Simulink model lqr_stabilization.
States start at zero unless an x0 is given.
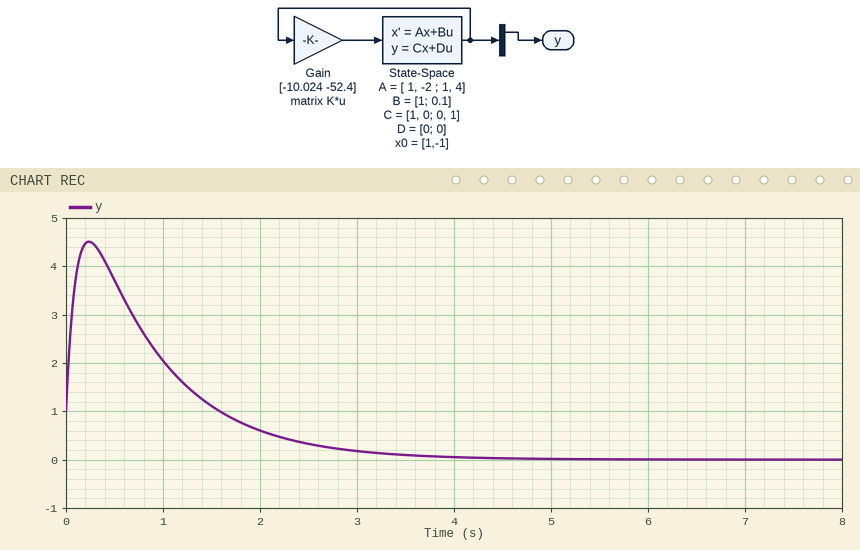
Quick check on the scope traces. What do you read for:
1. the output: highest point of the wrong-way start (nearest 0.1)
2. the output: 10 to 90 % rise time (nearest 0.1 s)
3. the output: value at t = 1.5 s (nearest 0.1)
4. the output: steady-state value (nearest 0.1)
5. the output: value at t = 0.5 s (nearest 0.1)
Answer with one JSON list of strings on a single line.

["4.5", "1.8 s", "1.1", "0.0", "3.7"]
